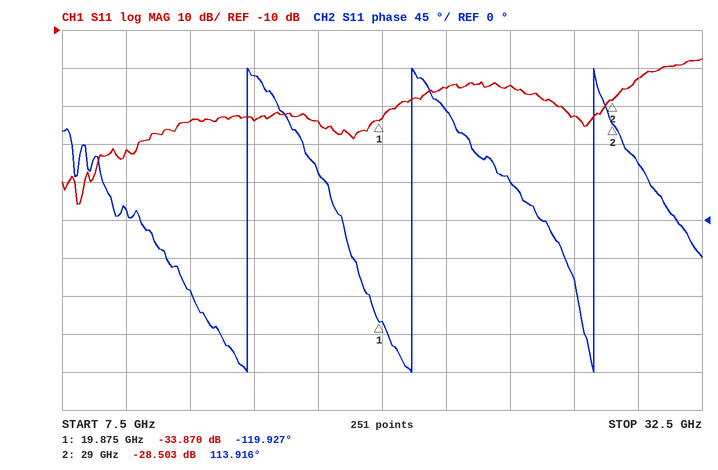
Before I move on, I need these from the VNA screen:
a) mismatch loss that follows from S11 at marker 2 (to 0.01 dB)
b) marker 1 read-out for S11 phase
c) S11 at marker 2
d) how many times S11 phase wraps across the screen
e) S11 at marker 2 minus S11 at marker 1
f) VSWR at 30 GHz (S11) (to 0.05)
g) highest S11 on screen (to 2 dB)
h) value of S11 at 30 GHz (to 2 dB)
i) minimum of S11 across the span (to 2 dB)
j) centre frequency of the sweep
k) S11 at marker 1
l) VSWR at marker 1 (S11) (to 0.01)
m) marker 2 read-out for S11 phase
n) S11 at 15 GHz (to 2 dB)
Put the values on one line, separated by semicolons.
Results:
0.01 dB; -119.927°; -28.503 dB; 3; 5.367 dB; 1.15; -18 dB; -22 dB; -56 dB; 20 GHz; -33.870 dB; 1.04; 113.916°; -34 dB
